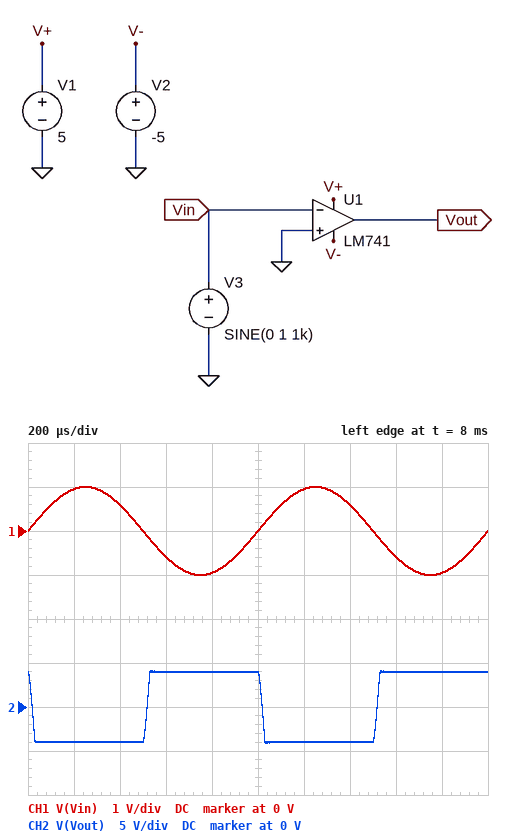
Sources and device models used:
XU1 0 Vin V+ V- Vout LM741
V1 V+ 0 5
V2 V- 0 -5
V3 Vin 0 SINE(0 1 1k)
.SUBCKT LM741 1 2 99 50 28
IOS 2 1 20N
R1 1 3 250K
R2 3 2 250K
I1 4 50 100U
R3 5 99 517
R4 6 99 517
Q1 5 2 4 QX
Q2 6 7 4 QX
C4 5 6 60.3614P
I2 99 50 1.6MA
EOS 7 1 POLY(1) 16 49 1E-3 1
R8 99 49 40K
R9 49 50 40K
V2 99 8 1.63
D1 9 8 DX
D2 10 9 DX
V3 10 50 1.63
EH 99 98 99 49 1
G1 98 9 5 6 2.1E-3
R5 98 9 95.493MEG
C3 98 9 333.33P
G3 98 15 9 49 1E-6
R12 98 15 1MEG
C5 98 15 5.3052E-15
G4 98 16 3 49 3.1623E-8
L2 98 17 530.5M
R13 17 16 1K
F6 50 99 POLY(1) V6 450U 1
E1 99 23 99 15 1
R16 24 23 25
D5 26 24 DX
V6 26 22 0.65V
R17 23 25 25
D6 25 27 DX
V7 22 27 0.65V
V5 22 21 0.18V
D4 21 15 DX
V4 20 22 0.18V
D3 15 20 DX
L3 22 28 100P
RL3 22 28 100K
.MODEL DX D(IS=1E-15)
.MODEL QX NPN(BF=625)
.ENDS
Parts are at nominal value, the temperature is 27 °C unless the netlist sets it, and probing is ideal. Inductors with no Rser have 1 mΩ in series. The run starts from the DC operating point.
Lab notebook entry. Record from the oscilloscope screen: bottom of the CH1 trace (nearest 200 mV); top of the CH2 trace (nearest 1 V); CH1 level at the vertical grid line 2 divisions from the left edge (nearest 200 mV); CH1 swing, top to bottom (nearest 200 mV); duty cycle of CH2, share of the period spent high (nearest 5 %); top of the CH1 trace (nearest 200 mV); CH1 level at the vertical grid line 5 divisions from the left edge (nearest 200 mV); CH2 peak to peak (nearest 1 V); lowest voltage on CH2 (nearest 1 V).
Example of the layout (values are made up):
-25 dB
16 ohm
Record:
-1.0 V
4 V
600 mV
2.0 V
50 %
1.0 V
0 V
8 V
-4 V
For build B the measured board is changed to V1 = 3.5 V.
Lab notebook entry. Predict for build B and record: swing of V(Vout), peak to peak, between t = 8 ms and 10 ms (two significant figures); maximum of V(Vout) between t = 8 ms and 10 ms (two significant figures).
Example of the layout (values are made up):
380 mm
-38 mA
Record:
6.6 V
2.5 V
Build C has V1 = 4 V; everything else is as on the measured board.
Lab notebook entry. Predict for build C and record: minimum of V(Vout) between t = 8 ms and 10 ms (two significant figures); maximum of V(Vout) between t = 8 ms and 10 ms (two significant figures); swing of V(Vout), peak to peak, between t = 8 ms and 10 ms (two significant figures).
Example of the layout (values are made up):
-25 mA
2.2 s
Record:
-4.0 V
3.0 V
7.1 V
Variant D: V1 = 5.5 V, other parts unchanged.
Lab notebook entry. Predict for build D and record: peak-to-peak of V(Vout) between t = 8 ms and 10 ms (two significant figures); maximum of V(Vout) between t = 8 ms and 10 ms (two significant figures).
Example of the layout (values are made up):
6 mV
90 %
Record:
8.6 V
4.5 V
